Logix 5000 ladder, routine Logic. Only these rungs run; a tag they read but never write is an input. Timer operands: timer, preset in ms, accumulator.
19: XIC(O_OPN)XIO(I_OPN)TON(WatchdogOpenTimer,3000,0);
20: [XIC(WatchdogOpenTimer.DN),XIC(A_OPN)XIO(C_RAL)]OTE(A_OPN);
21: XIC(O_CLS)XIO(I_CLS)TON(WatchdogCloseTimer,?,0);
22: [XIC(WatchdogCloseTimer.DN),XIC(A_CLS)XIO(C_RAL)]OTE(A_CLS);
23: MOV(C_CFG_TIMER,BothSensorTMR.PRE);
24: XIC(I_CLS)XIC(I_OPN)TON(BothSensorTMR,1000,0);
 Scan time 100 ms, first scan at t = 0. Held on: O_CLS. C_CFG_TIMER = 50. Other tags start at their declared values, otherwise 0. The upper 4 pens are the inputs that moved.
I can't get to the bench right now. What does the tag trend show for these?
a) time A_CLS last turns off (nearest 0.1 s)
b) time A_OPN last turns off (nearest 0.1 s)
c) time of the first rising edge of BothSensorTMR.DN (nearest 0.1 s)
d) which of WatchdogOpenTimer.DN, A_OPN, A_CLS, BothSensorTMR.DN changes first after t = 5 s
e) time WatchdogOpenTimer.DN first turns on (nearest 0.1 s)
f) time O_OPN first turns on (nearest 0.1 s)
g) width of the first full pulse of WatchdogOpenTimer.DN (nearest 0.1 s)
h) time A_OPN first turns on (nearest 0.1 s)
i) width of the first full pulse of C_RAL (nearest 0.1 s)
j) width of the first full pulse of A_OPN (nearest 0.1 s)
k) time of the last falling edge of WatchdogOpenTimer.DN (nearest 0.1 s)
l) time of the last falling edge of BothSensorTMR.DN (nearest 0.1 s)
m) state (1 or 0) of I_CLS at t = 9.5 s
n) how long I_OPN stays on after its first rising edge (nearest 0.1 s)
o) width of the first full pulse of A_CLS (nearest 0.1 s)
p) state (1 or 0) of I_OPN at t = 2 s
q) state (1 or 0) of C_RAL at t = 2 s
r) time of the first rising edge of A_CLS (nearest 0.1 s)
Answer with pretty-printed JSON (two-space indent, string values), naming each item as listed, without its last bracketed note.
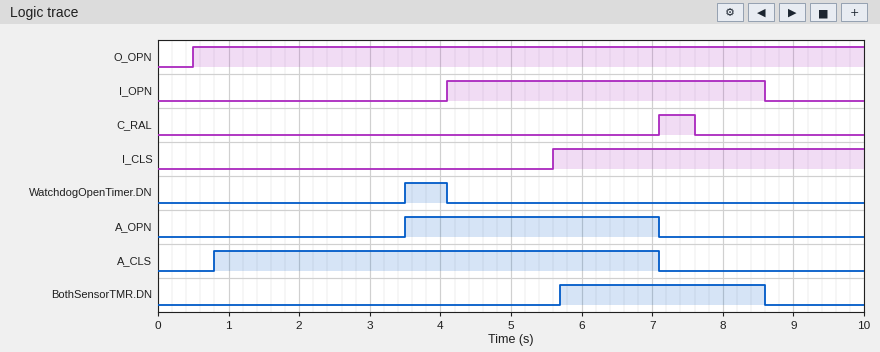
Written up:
{
  "time A_CLS last turns off": "7.1 s",
  "time A_OPN last turns off": "7.1 s",
  "time of the first rising edge of BothSensorTMR.DN": "5.7 s",
  "which of WatchdogOpenTimer.DN, A_OPN, A_CLS, BothSensorTMR.DN changes first after t = 5 s": "BothSensorTMR.DN",
  "time WatchdogOpenTimer.DN first turns on": "3.5 s",
  "time O_OPN first turns on": "0.5 s",
  "width of the first full pulse of WatchdogOpenTimer.DN": "0.6 s",
  "time A_OPN first turns on": "3.5 s",
  "width of the first full pulse of C_RAL": "0.5 s",
  "width of the first full pulse of A_OPN": "3.6 s",
  "time of the last falling edge of WatchdogOpenTimer.DN": "4.1 s",
  "time of the last falling edge of BothSensorTMR.DN": "8.6 s",
  "state (1 or 0) of I_CLS at t = 9.5 s": "1",
  "how long I_OPN stays on after its first rising edge": "4.5 s",
  "width of the first full pulse of A_CLS": "6.3 s",
  "state (1 or 0) of I_OPN at t = 2 s": "0",
  "state (1 or 0) of C_RAL at t = 2 s": "0",
  "time of the first rising edge of A_CLS": "0.8 s"
}
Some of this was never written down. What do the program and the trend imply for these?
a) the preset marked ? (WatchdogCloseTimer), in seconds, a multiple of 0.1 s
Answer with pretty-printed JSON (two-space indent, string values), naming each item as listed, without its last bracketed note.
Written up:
{
  "the preset marked ? (WatchdogCloseTimer), in seconds, a multiple of 0.1 s": "0.8 s"
}
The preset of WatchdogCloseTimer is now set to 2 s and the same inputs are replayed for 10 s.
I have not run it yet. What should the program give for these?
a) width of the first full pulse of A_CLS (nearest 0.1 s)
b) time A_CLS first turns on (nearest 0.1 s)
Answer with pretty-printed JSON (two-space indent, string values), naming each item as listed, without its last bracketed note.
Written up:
{
  "width of the first full pulse of A_CLS": "5.1 s",
  "time A_CLS first turns on": "2.0 s"
}
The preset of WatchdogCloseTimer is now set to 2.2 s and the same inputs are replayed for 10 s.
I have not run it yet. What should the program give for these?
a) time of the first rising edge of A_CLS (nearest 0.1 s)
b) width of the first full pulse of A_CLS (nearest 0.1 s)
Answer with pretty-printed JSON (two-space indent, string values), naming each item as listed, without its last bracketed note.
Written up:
{
  "time of the first rising edge of A_CLS": "2.2 s",
  "width of the first full pulse of A_CLS": "4.9 s"
}
